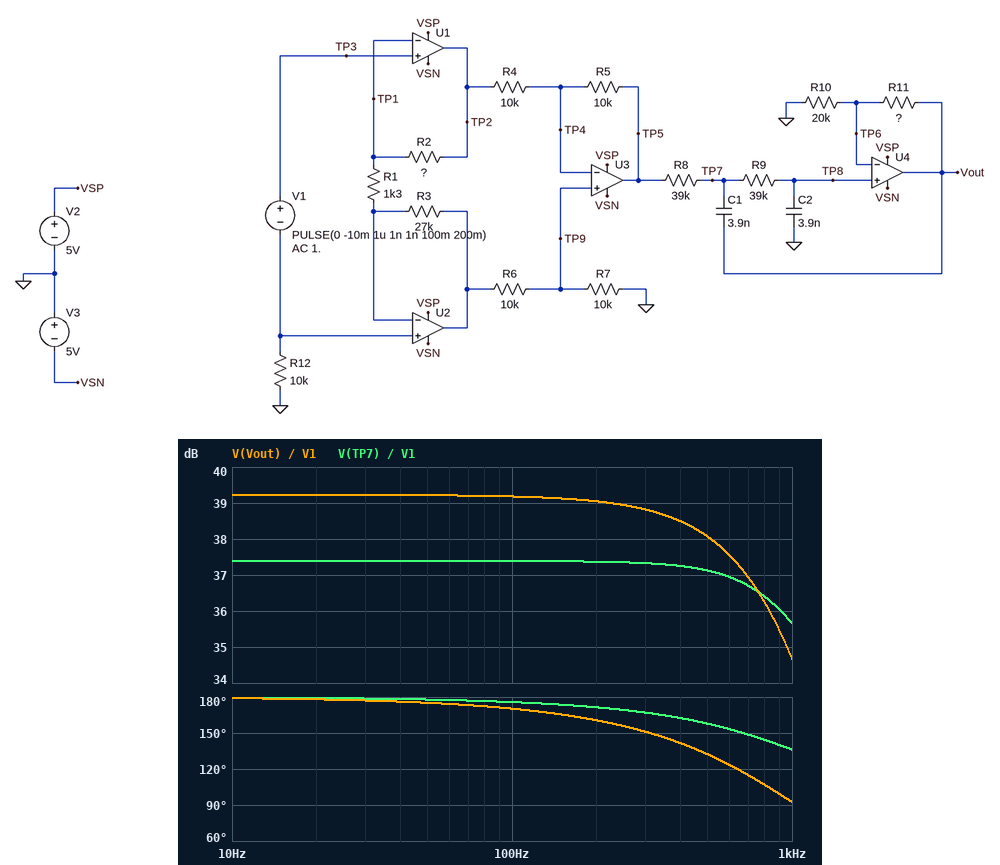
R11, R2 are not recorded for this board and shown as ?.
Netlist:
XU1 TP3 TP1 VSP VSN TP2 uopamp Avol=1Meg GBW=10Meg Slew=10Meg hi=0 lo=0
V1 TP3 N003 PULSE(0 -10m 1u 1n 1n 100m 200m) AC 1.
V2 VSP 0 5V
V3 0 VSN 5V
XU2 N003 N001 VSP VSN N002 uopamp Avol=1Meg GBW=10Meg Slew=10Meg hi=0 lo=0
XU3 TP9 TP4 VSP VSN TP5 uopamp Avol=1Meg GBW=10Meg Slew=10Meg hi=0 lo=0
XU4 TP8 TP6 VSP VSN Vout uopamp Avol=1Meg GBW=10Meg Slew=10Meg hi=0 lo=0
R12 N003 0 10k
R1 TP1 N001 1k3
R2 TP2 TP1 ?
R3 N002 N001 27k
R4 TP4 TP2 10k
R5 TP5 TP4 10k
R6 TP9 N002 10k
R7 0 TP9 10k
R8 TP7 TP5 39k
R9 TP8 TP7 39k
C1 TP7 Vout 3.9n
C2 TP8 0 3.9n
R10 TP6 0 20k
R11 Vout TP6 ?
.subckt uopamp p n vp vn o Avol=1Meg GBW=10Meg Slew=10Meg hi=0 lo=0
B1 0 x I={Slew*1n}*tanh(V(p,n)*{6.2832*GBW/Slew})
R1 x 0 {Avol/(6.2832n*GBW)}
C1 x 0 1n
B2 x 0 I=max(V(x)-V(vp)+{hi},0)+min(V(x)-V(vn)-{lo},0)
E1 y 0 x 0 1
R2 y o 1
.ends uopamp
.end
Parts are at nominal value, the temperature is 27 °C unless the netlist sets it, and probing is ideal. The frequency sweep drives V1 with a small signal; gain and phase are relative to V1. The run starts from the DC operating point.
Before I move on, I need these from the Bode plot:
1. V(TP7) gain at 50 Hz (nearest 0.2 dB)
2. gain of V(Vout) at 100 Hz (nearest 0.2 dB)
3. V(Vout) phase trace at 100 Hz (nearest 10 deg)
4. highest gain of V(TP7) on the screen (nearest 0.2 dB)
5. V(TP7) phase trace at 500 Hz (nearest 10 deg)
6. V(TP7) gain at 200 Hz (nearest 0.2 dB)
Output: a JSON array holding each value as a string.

["37.4 dB", "39.2 dB", "170 deg", "37.4 dB", "160 deg", "37.4 dB"]
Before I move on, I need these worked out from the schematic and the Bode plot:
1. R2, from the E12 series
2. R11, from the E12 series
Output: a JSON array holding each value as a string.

["68 kΩ", "4.7 kΩ"]
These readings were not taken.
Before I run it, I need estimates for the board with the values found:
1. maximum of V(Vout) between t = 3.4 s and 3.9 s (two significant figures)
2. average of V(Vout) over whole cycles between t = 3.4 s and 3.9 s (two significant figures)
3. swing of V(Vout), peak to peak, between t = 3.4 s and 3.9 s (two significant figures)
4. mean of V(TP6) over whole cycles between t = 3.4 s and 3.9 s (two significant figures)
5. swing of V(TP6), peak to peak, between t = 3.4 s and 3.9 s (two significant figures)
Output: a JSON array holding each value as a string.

["920 mV", "460 mV", "920 mV", "370 mV", "750 mV"]
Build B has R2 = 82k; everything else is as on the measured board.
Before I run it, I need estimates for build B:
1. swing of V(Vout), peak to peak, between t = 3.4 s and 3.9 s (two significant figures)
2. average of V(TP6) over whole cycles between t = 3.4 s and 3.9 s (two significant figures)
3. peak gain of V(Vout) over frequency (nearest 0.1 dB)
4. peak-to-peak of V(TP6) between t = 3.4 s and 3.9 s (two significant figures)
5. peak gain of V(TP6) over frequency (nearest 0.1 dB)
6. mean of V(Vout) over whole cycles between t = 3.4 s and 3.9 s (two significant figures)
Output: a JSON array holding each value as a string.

["1.1 V", "420 mV", "40.4 dB", "860 mV", "38.6 dB", "520 mV"]
